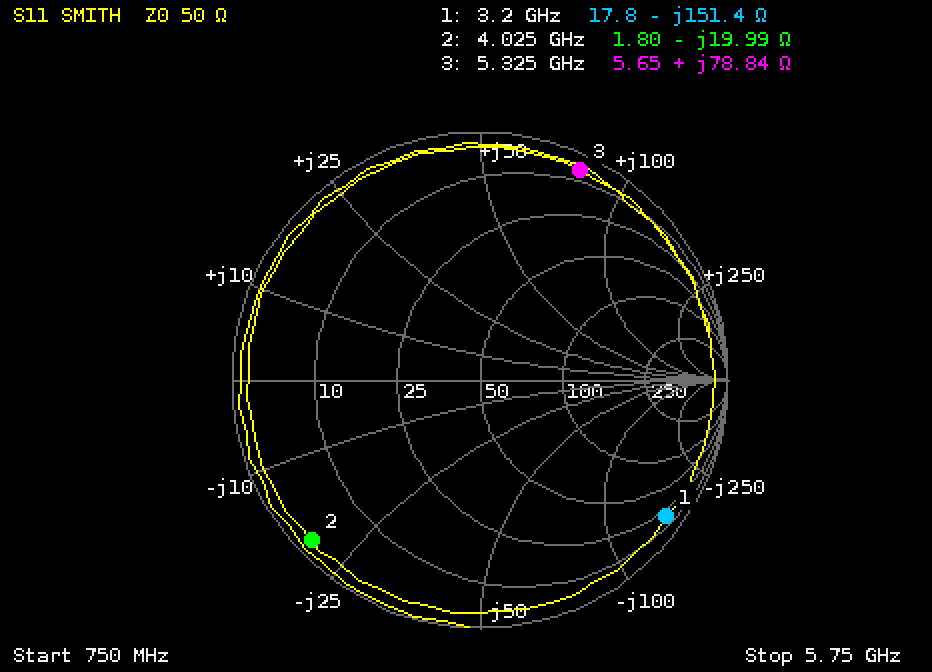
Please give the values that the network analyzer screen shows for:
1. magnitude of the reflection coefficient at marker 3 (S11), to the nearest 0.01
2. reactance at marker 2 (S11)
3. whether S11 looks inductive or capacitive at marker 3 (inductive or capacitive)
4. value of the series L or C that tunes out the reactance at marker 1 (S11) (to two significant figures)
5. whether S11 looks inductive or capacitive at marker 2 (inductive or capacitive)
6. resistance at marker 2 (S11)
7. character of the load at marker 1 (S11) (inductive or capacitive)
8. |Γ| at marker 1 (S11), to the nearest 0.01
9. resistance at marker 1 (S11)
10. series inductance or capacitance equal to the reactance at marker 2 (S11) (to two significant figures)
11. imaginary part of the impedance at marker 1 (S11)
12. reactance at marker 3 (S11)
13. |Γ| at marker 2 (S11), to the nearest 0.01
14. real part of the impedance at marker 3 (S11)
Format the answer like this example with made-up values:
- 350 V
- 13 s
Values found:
- 0.94
- -19.99 Ω
- inductive
- 7.5 nH
- capacitive
- 1.80 Ω
- capacitive
- 0.93
- 17.8 Ω
- 2.0 pF
- -151.4 Ω
- +78.84 Ω
- 0.94
- 5.65 Ω
